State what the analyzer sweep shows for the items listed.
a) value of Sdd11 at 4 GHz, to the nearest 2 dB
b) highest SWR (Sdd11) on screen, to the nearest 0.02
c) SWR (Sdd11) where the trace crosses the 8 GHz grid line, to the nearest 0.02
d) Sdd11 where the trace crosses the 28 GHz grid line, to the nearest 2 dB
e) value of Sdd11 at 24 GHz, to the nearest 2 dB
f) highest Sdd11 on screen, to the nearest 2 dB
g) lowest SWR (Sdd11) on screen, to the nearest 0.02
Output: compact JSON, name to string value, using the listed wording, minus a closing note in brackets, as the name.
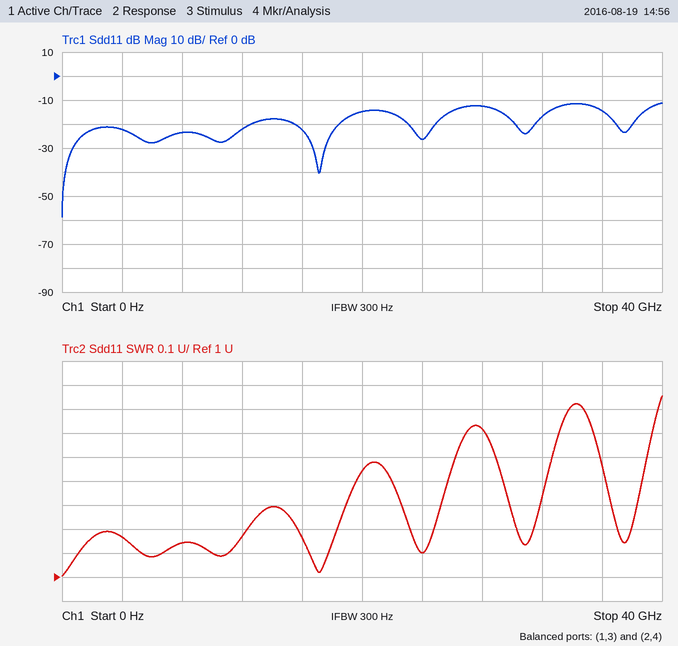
{"value of Sdd11 at 4 GHz, to the nearest 2 dB": "-22 dB", "highest SWR (Sdd11) on screen, to the nearest 0.02": "1.76", "SWR (Sdd11) where the trace crosses the 8 GHz grid line, to the nearest 0.02": "1.14", "Sdd11 where the trace crosses the 28 GHz grid line, to the nearest 2 dB": "-12 dB", "value of Sdd11 at 24 GHz, to the nearest 2 dB": "-26 dB", "highest Sdd11 on screen, to the nearest 2 dB": "-12 dB", "lowest SWR (Sdd11) on screen, to the nearest 0.02": "1.00"}
